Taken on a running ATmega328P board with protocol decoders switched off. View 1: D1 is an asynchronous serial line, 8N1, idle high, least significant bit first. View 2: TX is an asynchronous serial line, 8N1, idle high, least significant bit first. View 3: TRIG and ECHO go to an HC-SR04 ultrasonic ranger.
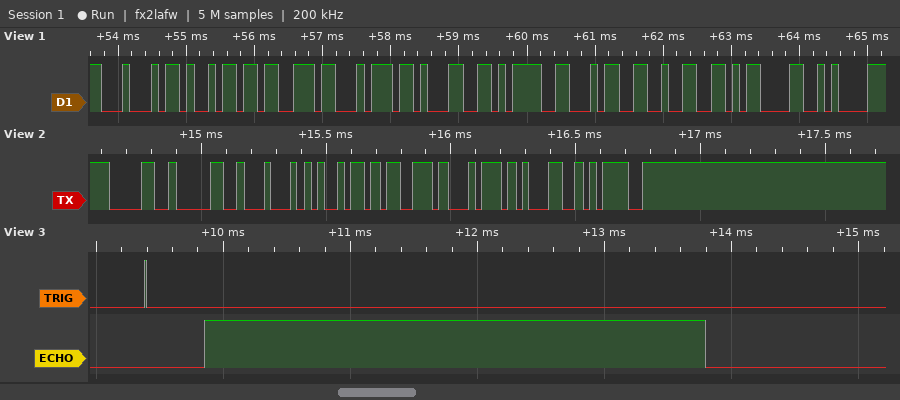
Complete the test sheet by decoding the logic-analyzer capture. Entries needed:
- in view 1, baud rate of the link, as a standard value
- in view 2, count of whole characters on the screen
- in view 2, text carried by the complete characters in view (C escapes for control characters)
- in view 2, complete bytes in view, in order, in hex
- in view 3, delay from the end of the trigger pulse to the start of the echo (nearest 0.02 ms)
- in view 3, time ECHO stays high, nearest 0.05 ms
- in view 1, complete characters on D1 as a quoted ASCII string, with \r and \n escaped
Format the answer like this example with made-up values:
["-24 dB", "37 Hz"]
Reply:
["9600 baud", "8", "\"00Dist1=\"", "30 30 44 69 73 74 31 3D", "0.46 ms", "3.95 ms", "\"Dist1=42\\r\\n\""]
